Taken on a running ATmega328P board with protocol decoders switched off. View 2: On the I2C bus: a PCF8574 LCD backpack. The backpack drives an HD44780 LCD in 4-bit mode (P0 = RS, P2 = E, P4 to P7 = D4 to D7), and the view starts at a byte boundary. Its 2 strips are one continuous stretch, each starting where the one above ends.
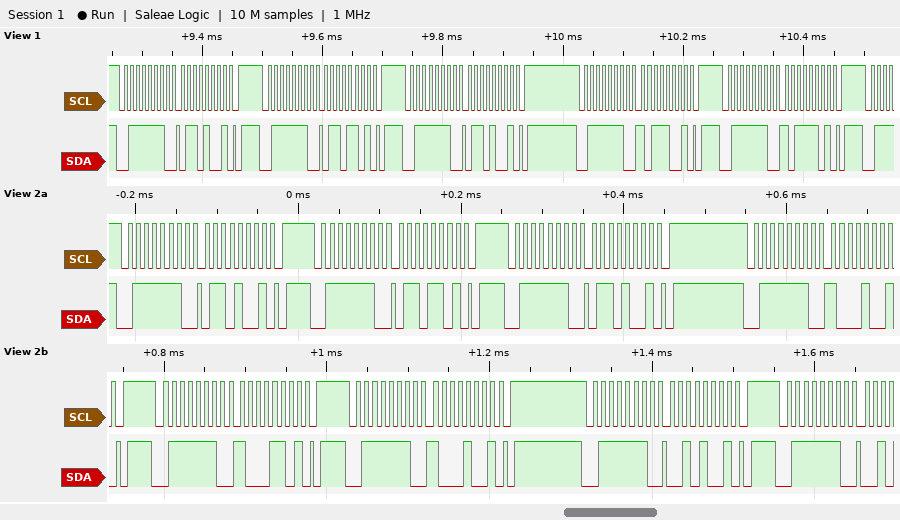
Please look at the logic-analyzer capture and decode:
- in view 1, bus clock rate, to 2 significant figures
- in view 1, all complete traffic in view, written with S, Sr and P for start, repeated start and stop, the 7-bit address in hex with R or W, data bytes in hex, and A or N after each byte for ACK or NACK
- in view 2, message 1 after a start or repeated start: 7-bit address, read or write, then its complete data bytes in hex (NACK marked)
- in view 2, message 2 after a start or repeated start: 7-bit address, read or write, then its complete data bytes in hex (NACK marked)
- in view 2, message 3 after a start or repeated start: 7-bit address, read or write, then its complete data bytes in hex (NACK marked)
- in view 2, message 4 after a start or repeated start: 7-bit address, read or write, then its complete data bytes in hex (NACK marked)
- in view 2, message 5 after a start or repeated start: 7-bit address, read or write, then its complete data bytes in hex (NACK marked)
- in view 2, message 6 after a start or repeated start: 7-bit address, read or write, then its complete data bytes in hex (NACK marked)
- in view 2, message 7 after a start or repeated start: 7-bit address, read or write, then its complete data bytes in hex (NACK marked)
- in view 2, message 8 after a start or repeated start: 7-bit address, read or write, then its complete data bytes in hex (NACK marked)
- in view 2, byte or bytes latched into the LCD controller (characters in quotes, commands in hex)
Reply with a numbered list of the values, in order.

1. 100 kHz
2. S 3FW A 69 A P S 3FW A 6D A P S 3FW A 69 A P S 3FW A B9 A P S 3FW A BD A P
3. 0x3F write: 69
4. 0x3F write: 6D
5. 0x3F write: 69
6. 0x3F write: 89
7. 0x3F write: 8D
8. 0x3F write: 89
9. 0x3F write: 29
10. 0x3F write
11. 'h'
